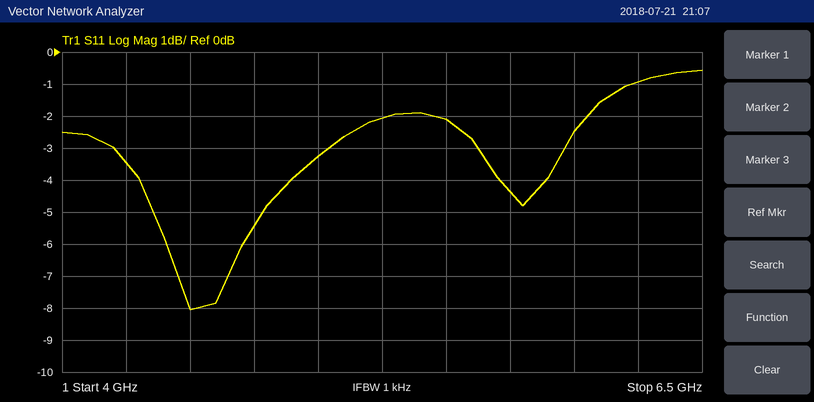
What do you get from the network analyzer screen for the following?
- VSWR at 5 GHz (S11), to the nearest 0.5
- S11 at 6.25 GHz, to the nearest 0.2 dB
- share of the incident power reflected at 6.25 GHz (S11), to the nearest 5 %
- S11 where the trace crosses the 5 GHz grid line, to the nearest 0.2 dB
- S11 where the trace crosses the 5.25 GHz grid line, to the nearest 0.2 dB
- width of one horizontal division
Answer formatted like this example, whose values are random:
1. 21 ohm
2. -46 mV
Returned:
1. 5.5
2. -1.0 dB
3. 80 %
4. -3.2 dB
5. -2.0 dB
6. 250 MHz
